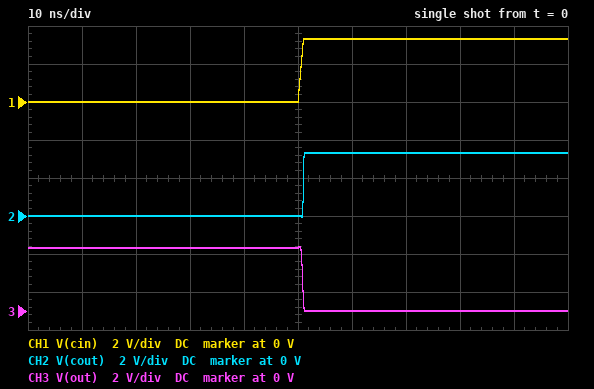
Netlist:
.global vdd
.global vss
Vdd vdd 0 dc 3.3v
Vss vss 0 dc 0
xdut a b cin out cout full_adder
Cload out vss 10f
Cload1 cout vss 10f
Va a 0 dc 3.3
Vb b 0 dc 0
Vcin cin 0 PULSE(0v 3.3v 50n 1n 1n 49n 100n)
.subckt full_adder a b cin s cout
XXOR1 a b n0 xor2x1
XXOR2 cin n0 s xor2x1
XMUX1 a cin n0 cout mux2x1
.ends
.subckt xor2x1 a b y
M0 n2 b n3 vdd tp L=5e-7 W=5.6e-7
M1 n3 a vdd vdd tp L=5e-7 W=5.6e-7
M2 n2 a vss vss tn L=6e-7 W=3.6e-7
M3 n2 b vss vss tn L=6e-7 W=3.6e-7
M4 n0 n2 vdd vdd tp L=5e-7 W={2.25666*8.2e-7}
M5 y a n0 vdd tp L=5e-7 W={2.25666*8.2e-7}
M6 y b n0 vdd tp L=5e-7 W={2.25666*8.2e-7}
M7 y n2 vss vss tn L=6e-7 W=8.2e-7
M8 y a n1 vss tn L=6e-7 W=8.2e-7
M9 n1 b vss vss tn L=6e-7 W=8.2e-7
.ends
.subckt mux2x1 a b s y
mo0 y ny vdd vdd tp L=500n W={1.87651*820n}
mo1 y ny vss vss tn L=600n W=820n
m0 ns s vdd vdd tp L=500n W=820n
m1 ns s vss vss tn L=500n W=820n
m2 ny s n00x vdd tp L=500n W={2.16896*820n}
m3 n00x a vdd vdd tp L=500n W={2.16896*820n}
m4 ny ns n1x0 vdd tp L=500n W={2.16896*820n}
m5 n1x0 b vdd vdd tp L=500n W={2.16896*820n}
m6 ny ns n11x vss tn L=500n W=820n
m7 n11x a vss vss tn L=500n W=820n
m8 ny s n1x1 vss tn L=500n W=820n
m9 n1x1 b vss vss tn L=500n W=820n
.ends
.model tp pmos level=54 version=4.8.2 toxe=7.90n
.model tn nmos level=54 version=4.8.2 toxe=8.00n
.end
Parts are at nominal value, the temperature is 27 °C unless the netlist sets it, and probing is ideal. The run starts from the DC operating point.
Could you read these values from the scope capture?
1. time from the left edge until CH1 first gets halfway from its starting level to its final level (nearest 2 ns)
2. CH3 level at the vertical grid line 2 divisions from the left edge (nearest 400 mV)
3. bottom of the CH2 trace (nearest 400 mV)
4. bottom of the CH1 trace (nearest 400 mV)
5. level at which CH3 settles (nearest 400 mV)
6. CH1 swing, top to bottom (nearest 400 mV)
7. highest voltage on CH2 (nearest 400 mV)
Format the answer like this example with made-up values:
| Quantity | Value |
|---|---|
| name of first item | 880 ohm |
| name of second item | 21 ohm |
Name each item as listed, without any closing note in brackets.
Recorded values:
| Quantity | Value |
|---|---|
| time from the left edge until CH1 first gets halfway from its starting level to its final level | 50 ns |
| CH3 level at the vertical grid line 2 divisions from the left edge | 3.2 V |
| bottom of the CH2 trace | 0 V |
| bottom of the CH1 trace | 0 V |
| level at which CH3 settles | 0 V |
| CH1 swing, top to bottom | 3.2 V |
| highest voltage on CH2 | 3.2 V |
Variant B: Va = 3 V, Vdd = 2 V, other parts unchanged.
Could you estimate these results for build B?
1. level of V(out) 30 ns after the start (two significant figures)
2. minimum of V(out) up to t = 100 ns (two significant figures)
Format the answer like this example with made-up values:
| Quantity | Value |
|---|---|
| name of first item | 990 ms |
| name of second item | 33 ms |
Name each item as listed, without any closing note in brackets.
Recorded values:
| Quantity | Value |
|---|---|
| level of V(out) 30 ns after the start | 2.0 V |
| minimum of V(out) up to t = 100 ns | -4.7 mV |
